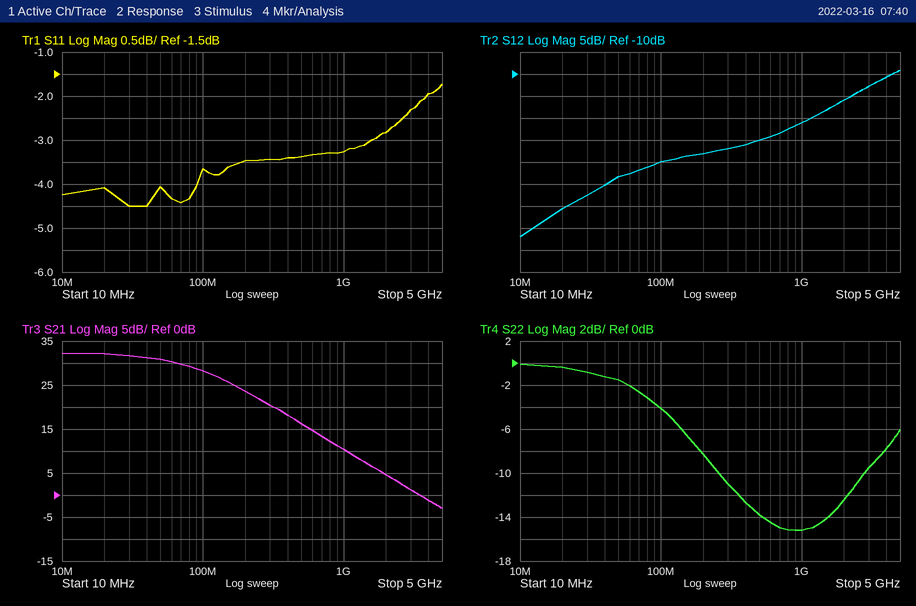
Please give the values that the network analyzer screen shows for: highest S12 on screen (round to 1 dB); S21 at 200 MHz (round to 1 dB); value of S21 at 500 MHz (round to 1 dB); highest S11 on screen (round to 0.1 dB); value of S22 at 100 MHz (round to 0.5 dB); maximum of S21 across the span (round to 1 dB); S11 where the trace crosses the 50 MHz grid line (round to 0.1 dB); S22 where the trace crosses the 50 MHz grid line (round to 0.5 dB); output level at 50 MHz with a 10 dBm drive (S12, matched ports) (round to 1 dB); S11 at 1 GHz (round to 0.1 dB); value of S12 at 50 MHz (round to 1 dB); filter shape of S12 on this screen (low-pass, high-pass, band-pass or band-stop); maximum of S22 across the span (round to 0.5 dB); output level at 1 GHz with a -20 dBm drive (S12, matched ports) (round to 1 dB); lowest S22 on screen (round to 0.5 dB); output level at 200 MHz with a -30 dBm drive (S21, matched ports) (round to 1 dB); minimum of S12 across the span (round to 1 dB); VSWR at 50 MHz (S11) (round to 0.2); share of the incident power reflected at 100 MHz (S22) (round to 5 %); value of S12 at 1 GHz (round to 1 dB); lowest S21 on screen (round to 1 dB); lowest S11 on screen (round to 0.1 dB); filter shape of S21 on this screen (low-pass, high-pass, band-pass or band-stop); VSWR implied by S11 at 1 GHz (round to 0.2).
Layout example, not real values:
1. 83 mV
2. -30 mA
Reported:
1. -9 dB
2. 24 dB
3. 16 dB
4. -1.7 dB
5. -4.0 dB
6. 32 dB
7. -4.1 dB
8. -1.5 dB
9. -23 dBm
10. -3.3 dB
11. -33 dB
12. high-pass
13. 0.0 dB
14. -41 dBm
15. -15.0 dB
16. -6 dBm
17. -47 dB
18. 4.4
19. 40 %
20. -21 dB
21. -3 dB
22. -4.5 dB
23. low-pass
24. 5.4
